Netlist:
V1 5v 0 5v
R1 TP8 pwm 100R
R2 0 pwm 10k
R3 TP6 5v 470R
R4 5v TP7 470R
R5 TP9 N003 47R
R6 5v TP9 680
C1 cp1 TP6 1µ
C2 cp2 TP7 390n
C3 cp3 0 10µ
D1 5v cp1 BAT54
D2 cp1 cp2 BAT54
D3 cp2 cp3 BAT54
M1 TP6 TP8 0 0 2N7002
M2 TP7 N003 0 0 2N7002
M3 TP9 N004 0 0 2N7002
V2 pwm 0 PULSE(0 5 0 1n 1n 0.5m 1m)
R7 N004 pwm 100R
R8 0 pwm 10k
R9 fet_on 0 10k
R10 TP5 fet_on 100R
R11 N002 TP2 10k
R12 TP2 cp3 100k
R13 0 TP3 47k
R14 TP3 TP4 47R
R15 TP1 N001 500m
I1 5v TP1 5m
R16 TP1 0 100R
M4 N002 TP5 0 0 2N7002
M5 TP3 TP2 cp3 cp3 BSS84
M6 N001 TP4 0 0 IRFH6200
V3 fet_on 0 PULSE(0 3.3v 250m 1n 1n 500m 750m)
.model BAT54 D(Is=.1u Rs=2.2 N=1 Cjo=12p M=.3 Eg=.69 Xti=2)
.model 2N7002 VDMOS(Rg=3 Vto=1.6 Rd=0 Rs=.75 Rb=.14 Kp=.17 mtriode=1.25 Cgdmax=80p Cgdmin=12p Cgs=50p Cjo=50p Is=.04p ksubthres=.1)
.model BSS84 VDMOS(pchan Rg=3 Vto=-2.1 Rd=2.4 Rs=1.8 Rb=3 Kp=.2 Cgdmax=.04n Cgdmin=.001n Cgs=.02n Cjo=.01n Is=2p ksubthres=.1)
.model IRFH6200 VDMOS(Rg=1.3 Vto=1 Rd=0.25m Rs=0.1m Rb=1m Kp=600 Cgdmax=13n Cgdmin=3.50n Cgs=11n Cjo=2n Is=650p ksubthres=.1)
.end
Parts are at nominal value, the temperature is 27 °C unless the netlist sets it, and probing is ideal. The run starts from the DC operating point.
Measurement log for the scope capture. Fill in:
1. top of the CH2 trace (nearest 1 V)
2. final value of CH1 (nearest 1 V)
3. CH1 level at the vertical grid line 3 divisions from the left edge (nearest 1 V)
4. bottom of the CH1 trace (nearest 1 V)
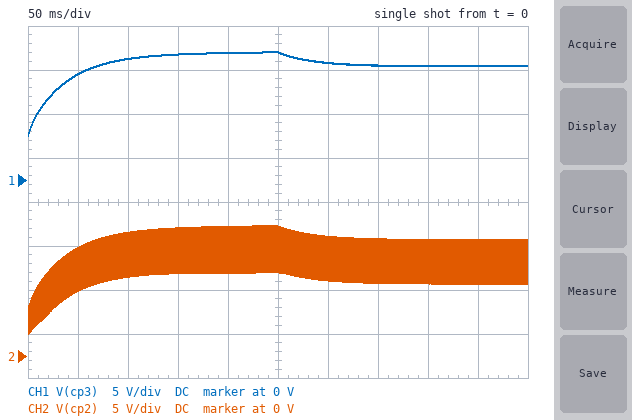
15 V
13 V
14 V
5 V
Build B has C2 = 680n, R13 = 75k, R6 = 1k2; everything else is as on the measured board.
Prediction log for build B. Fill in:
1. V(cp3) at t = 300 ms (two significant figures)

14 V
